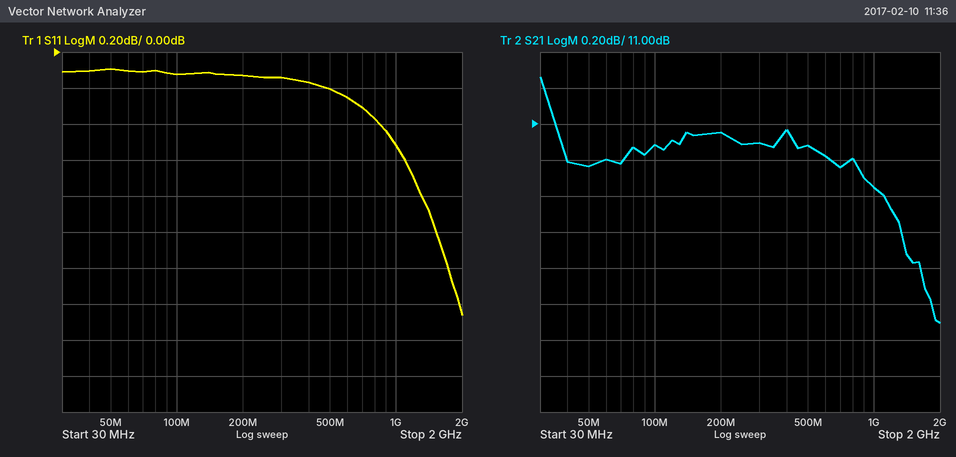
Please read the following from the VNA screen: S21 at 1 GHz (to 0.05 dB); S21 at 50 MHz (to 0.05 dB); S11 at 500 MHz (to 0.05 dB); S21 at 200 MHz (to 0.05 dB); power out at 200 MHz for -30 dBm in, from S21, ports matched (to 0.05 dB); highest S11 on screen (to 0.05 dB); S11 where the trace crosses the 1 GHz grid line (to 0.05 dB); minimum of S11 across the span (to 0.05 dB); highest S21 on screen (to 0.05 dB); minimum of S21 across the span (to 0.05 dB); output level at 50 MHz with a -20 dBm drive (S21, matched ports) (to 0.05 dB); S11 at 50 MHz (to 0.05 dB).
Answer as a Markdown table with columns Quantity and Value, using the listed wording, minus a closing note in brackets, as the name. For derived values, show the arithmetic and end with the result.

| Quantity | Value |
|---|---|
| S21 at 1 GHz | 10.65 dB |
| S21 at 50 MHz | 10.75 dB |
| S11 at 500 MHz | -0.20 dB |
| S21 at 200 MHz | 10.95 dB |
| power out at 200 MHz for -30 dBm in, from S21, ports matched | -30 dBm + (10.95 dB) = -19.05 dBm |
| highest S11 on screen | -0.10 dB |
| S11 where the trace crosses the 1 GHz grid line | -0.50 dB |
| minimum of S11 across the span | -1.45 dB |
| highest S21 on screen | 11.25 dB |
| minimum of S21 across the span | 9.90 dB |
| output level at 50 MHz with a -20 dBm drive (S21, matched ports) | -20 dBm + (10.75 dB) = -9.25 dBm |
| S11 at 50 MHz | -0.10 dB |
